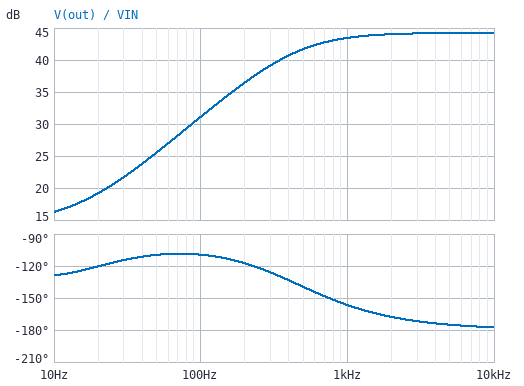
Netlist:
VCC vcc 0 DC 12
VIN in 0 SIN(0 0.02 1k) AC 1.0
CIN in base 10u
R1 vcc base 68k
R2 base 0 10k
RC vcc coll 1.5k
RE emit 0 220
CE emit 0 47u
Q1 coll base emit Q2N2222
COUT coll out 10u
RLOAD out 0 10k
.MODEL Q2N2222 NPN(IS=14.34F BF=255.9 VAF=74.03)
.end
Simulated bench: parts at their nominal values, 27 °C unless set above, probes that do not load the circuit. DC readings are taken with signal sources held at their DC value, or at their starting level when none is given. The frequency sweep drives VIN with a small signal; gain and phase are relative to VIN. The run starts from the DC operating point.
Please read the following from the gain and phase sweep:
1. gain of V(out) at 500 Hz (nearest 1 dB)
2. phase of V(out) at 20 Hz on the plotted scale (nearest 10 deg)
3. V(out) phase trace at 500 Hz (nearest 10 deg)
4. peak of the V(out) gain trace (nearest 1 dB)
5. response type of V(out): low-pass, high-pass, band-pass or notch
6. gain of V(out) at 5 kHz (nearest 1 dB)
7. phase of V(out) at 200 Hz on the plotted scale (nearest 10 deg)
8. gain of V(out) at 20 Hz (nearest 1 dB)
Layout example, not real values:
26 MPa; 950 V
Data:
42 dB; -120 deg; -140 deg; 44 dB; high-pass; 44 dB; -120 deg; 19 dB
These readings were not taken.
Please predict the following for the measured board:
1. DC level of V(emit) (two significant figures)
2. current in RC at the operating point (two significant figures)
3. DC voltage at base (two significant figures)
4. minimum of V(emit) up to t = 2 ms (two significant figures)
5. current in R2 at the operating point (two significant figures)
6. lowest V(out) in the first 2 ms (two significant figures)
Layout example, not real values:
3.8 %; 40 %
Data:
750 mV; 3.4 mA; 1.4 V; 750 mV; 140 µA; -3.3 V
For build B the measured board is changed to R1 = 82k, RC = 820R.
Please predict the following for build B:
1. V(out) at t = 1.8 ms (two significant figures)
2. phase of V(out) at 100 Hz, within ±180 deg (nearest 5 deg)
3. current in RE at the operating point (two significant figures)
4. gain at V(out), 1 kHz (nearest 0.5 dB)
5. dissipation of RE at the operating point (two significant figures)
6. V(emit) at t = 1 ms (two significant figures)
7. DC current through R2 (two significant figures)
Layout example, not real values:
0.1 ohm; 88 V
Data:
990 mV; -115 deg; 2.5 mA; 36.5 dB; 1.4 mW; 560 mV; 120 µA
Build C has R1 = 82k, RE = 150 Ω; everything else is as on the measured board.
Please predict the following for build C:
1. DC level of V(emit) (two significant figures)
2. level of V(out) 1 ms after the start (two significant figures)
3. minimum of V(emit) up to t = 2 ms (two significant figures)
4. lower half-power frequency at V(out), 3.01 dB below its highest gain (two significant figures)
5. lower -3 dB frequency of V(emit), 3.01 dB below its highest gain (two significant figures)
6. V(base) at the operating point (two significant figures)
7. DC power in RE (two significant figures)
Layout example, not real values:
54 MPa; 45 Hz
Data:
520 mV; -790 mV; 510 mV; 460 Hz; 2.1 Hz; 1.2 V; 1.8 mW
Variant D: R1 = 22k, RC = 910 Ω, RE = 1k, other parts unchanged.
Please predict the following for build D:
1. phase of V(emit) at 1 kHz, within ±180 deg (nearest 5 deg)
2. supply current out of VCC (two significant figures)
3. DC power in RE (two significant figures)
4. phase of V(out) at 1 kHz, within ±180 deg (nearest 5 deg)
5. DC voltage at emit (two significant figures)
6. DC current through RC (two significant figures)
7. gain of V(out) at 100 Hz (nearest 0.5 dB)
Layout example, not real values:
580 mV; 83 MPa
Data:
-70 deg; 3.4 mA; 9.0 mW; -160 deg; 3.0 V; 3.0 mA; 27.5 dB
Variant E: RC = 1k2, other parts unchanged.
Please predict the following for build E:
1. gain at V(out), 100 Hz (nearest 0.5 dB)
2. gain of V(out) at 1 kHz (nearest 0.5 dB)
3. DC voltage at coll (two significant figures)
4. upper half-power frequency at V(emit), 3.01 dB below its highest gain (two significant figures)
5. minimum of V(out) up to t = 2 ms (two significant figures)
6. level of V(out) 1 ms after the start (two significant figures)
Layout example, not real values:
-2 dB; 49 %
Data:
29.5 dB; 42.0 dB; 7.9 V; 460 Hz; -2.7 V; -650 mV
